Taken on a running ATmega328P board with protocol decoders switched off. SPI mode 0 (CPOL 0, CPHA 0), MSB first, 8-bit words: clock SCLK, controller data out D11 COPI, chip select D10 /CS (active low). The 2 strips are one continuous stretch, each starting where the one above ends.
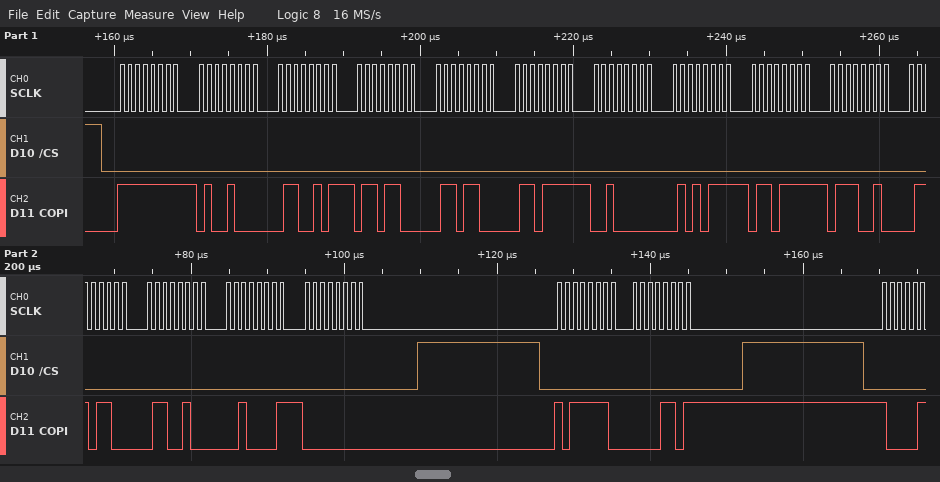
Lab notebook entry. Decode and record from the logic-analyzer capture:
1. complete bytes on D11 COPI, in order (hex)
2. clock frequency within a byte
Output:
0xFF 0x48 0x65 0x6C 0x6C 0x6F 0x20 0x57 0x6F 0x72 0x6C 0x64 0x21 0x00 0xBE 0x0D
1 MHz
